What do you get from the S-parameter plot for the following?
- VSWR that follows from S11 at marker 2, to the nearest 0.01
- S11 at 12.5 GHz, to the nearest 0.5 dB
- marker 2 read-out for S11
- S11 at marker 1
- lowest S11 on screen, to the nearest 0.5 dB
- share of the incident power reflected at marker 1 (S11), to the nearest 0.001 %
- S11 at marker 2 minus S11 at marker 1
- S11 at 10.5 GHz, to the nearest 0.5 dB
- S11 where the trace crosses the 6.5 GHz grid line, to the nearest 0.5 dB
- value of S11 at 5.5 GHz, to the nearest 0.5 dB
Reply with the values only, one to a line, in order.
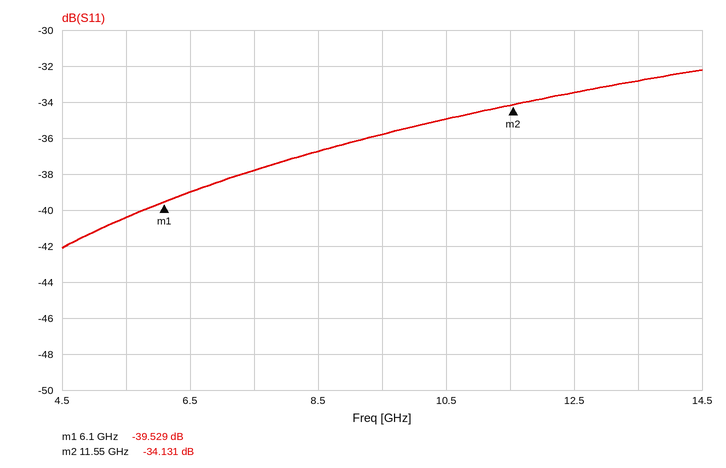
1.04
-33.5 dB
-34.131 dB
-39.529 dB
-42.0 dB
0.011 %
5.398 dB
-35.0 dB
-39.0 dB
-40.5 dB
